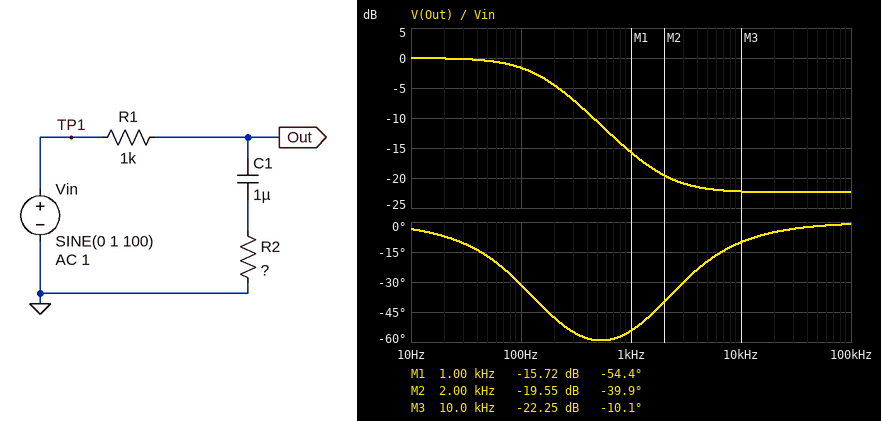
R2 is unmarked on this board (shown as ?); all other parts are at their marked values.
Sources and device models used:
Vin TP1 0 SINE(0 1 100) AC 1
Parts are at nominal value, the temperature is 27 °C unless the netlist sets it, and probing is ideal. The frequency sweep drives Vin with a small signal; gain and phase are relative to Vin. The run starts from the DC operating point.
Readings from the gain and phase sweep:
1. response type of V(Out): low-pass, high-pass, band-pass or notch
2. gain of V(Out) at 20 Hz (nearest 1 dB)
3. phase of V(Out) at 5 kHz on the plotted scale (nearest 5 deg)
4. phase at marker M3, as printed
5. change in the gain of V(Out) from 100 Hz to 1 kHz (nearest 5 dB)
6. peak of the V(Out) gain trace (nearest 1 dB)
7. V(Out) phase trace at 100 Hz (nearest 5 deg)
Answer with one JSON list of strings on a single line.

["low-pass", "0 dB", "-20 deg", "-10.1 deg", "-15 dB", "0 dB", "-30 deg"]
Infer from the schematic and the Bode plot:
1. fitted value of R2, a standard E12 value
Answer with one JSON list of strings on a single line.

["82 Ω"]
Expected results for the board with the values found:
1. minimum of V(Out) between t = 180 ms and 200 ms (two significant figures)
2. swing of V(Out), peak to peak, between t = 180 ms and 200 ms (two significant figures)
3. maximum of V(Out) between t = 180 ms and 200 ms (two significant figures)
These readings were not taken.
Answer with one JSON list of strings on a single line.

["-830 mV", "1.7 V", "830 mV"]
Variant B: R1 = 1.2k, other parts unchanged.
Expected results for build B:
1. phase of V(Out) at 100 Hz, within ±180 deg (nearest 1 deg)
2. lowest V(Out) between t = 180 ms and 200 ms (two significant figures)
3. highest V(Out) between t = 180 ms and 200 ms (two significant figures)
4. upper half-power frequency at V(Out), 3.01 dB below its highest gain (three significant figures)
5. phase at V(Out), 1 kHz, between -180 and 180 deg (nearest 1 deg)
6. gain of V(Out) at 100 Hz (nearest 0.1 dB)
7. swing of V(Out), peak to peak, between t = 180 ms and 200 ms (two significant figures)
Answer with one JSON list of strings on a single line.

["-36 deg", "-780 mV", "780 mV", "125 Hz", "-56 deg", "-2.2 dB", "1.6 V"]
